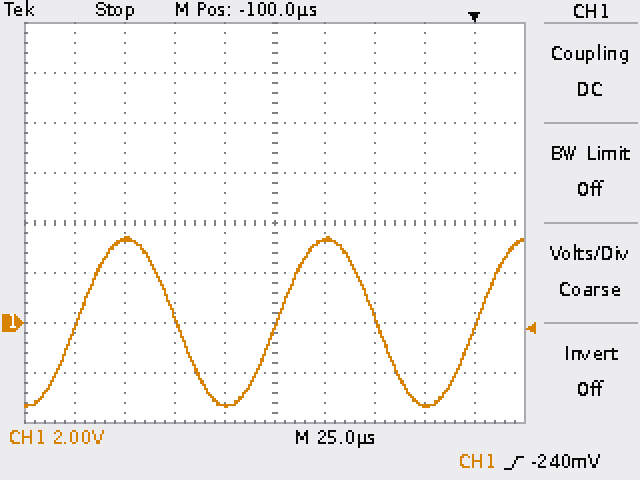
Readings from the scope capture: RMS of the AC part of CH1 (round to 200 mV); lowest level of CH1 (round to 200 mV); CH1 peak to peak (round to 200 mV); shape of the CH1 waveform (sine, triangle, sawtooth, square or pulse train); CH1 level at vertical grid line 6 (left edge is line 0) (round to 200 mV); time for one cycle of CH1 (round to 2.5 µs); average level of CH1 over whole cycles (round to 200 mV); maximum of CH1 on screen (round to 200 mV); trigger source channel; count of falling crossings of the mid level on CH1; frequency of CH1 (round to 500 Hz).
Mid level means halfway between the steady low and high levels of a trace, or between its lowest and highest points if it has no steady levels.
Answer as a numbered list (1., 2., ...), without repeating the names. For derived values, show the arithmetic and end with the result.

1. 6.8 V / (2√2) ≈ 2.4 V
2. -3.4 V
3. 3.4 V − (-3.4 V) = 6.8 V
4. sine
5. 3.4 V
6. 100.0 µs
7. (3.4 V + (-3.4 V)) / 2 ≈ 0.0 V
8. 3.4 V
9. CH1
10. 2
11. 1 / 100.0 µs ≈ 10.0 kHz
